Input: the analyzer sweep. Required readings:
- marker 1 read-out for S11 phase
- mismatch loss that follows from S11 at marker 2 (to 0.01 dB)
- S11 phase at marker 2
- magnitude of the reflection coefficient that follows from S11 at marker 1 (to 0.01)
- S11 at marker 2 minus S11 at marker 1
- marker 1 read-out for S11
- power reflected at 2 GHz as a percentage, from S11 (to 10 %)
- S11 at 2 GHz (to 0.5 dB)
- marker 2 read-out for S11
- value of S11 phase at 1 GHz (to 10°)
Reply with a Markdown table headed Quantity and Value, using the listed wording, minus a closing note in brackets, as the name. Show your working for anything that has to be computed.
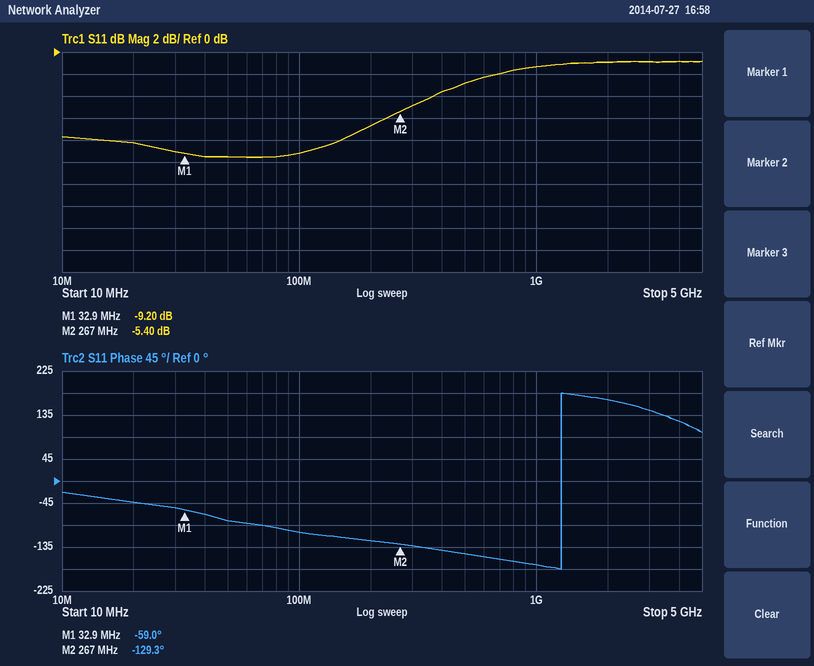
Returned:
| Quantity | Value |
|---|---|
| marker 1 read-out for S11 phase | -59.0° |
| mismatch loss that follows from S11 at marker 2 | −10 log10(1 − 10^(-5.4/10)) ≈ 1.48 dB |
| S11 phase at marker 2 | -129.3° |
| magnitude of the reflection coefficient that follows from S11 at marker 1 | 10^(-9.2/20) ≈ 0.35 |
| S11 at marker 2 minus S11 at marker 1 | -5.4 − (-9.2) = 3.80 dB |
| marker 1 read-out for S11 | -9.20 dB |
| power reflected at 2 GHz as a percentage, from S11 | 10^(-1/10) ≈ 79.4 %, so 80 % to the nearest 10 % |
| S11 at 2 GHz | -1.0 dB |
| marker 2 read-out for S11 | -5.40 dB |
| value of S11 phase at 1 GHz | -170° |
